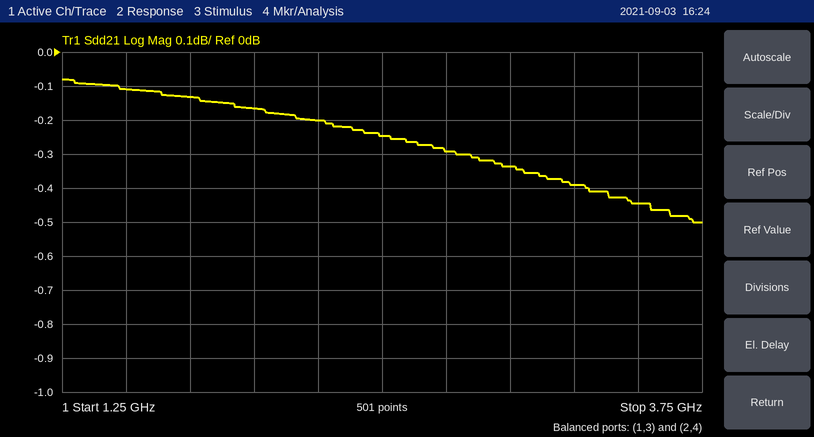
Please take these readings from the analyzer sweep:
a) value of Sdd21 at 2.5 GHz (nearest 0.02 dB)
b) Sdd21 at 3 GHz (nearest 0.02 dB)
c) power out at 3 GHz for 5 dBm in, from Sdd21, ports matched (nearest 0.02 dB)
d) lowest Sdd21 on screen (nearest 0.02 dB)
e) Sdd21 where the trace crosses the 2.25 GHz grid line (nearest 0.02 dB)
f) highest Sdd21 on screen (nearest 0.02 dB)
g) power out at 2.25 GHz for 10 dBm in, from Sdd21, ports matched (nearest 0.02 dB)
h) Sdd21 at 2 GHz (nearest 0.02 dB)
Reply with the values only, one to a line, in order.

-0.24 dB
-0.34 dB
4.66 dBm
-0.50 dB
-0.20 dB
-0.08 dB
9.80 dBm
-0.16 dB
